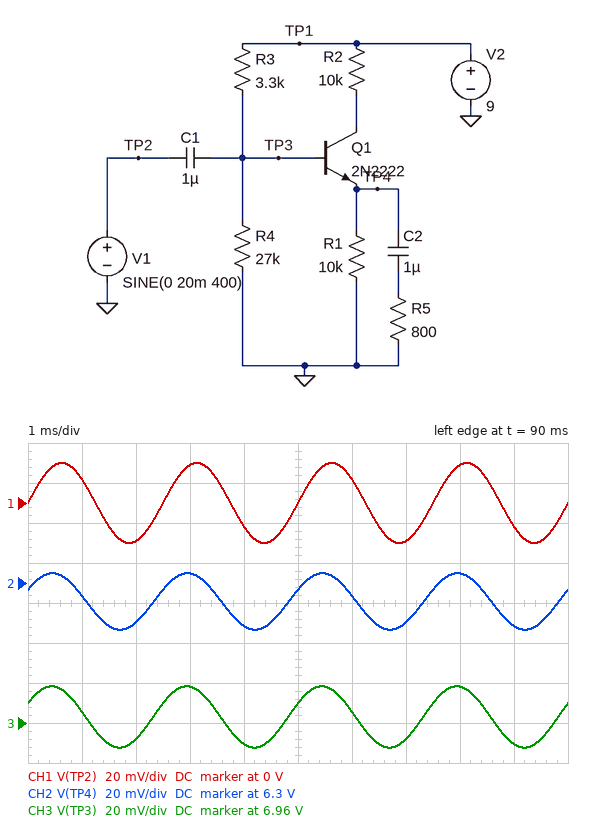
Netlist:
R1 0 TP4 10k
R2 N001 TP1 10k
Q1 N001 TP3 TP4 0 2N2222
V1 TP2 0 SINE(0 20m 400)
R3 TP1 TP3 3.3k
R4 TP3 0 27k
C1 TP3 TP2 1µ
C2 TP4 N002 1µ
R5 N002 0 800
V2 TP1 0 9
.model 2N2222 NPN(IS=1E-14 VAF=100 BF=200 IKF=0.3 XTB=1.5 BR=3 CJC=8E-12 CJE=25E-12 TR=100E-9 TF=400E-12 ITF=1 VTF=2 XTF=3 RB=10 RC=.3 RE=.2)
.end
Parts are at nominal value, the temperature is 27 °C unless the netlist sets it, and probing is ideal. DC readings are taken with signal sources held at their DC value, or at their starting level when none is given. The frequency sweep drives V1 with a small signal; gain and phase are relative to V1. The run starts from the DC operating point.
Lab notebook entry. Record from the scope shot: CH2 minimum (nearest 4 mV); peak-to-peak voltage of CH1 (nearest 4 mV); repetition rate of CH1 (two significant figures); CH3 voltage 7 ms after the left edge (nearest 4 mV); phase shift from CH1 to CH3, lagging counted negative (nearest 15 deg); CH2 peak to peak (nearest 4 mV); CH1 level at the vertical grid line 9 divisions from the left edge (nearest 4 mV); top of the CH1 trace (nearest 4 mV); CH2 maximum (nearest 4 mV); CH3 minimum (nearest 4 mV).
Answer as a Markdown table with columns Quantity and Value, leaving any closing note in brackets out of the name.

| Quantity | Value |
|---|---|
| CH2 minimum | 6.276 V |
| peak-to-peak voltage of CH1 | 40 mV |
| repetition rate of CH1 | 400 Hz |
| CH3 voltage 7 ms after the left edge | 6.952 V |
| phase shift from CH1 to CH3, lagging counted negative | 30 deg |
| CH2 peak to peak | 28 mV |
| CH1 level at the vertical grid line 9 divisions from the left edge | -12 mV |
| top of the CH1 trace | 20 mV |
| CH2 maximum | 6.304 V |
| CH3 minimum | 6.948 V |
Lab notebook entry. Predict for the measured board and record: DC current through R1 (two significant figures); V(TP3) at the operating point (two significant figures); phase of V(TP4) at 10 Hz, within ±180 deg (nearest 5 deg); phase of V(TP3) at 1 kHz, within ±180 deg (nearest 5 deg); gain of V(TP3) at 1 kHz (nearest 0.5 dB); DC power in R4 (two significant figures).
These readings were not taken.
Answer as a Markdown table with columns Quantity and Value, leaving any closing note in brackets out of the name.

| Quantity | Value |
|---|---|
| DC current through R1 | 630 µA |
| V(TP3) at the operating point | 7.0 V |
| phase of V(TP4) at 10 Hz, within ±180 deg | 75 deg |
| phase of V(TP3) at 1 kHz, within ±180 deg | 15 deg |
| gain of V(TP3) at 1 kHz | -0.5 dB |
| DC power in R4 | 1.8 mW |
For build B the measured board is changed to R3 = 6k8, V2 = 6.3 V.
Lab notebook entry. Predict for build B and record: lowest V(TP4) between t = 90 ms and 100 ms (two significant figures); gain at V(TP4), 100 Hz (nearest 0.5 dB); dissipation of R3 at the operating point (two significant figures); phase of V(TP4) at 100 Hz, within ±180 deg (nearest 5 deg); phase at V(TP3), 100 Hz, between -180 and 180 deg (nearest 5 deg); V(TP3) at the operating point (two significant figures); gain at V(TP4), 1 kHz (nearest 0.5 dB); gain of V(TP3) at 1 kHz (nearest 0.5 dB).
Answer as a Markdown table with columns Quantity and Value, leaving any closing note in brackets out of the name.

| Quantity | Value |
|---|---|
| lowest V(TP4) between t = 90 ms and 100 ms | 3.7 V |
| gain at V(TP4), 100 Hz | -6.5 dB |
| dissipation of R3 at the operating point | 540 µW |
| phase of V(TP4) at 100 Hz, within ±180 deg | 25 deg |
| phase at V(TP3), 100 Hz, between -180 and 180 deg | 30 deg |
| V(TP3) at the operating point | 4.4 V |
| gain at V(TP4), 1 kHz | -2.0 dB |
| gain of V(TP3) at 1 kHz | -0.5 dB |
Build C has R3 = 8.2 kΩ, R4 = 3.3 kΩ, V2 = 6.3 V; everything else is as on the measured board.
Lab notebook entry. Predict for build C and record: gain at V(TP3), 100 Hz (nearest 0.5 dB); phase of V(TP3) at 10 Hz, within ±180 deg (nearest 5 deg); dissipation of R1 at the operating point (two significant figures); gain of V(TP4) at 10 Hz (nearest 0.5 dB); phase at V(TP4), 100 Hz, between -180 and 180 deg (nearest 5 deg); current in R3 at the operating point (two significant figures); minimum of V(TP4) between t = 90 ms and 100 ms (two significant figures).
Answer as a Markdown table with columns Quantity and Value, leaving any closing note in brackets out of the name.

| Quantity | Value |
|---|---|
| gain at V(TP3), 100 Hz | -1.5 dB |
| phase of V(TP3) at 10 Hz, within ±180 deg | 80 deg |
| dissipation of R1 at the operating point | 150 µW |
| gain of V(TP4) at 10 Hz | -17.0 dB |
| phase at V(TP4), 100 Hz, between -180 and 180 deg | 30 deg |
| current in R3 at the operating point | 550 µA |
| minimum of V(TP4) between t = 90 ms and 100 ms | 1.2 V |
